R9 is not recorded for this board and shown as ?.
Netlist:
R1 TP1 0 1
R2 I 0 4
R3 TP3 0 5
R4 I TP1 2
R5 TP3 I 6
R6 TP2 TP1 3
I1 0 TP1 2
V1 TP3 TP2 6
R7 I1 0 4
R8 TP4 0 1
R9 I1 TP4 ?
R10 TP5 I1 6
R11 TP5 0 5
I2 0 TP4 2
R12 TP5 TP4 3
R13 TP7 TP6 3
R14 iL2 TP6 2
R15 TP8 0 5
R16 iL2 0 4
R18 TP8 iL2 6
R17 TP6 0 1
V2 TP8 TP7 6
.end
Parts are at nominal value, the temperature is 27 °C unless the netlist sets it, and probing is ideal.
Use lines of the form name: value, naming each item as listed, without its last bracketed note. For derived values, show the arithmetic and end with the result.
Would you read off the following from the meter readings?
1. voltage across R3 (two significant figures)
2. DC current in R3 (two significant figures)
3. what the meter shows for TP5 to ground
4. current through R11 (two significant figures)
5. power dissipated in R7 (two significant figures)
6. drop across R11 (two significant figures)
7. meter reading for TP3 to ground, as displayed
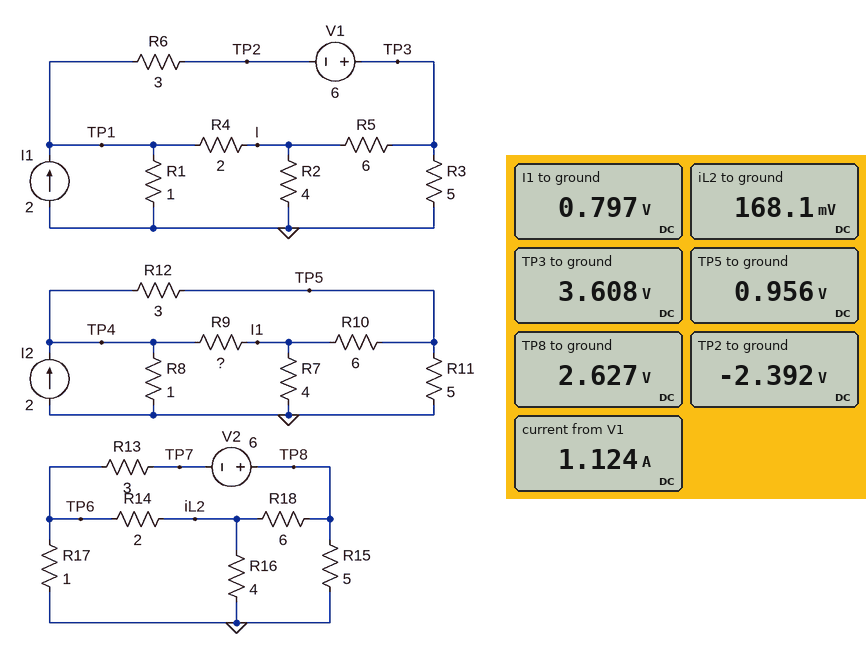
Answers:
voltage across R3: 3.608 V = 3.6 V
DC current in R3: (3.608 V) / 5 Ω = 720 mA
what the meter shows for TP5 to ground: 0.956 V
current through R11: (956 mV) / 5 Ω = 190 mA
power dissipated in R7: (797 mV)^2 / 4 Ω = 160 mW
drop across R11: 956 mV = 960 mV
meter reading for TP3 to ground, as displayed: 3.608 V
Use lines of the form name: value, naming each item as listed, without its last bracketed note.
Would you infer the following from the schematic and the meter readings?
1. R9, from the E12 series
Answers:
R9, from the E12 series: 4.7 Ω
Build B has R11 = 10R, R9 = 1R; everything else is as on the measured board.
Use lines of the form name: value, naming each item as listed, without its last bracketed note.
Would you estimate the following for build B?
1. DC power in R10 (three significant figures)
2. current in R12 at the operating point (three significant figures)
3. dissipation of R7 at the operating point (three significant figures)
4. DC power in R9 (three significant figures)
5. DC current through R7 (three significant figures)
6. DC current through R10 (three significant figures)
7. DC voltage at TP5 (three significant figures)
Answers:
DC power in R10: 168 µW
current in R12 at the operating point: 116 mA
dissipation of R7 at the operating point: 390 mW
DC power in R9: 101 mW
DC current through R7: 312 mA
DC current through R10: 5.29 mA
DC voltage at TP5: 1.22 V
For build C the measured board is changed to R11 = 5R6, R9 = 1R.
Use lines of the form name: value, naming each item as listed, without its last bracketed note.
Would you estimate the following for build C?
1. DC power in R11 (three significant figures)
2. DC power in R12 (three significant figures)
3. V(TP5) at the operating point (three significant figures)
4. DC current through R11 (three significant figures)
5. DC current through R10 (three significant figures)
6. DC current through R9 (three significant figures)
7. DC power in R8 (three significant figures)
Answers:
DC power in R11: 192 mW
DC power in R12: 76.4 mW
V(TP5) at the operating point: 1.04 V
DC current through R11: 185 mA
DC current through R10: 25.8 mA
DC current through R9: 324 mA
DC power in R8: 2.30 W
